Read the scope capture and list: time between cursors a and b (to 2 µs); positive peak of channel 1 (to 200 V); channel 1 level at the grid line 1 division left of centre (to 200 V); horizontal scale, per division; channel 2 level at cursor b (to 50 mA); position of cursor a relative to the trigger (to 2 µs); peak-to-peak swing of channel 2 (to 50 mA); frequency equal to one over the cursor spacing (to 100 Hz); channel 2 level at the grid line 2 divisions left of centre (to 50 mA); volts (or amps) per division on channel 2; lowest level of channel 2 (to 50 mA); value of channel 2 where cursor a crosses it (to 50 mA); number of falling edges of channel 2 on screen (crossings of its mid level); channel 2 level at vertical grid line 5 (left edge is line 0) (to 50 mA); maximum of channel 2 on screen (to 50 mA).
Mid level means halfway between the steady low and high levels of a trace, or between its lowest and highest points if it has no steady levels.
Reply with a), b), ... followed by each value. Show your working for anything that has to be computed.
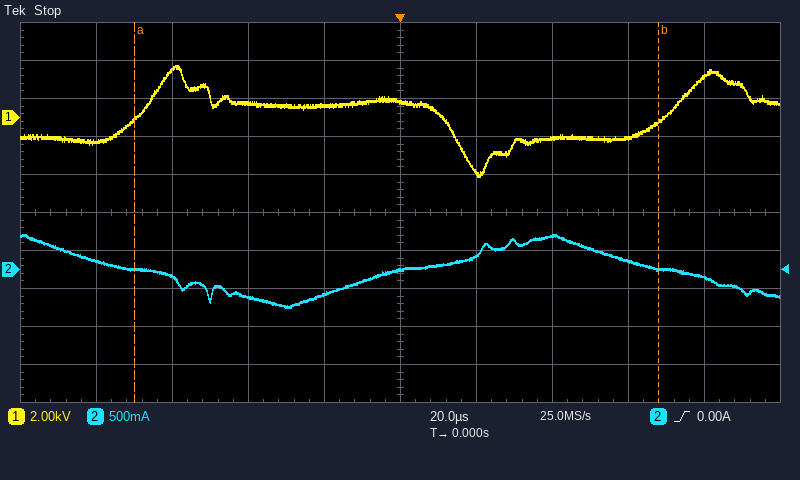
a) 138 µs
b) 2.8 kV
c) 600 V
d) 20 µs
e) 0 mA
f) -70 µs
g) 450 mA − (-500 mA) = 950 mA
h) 1 / 138 µs ≈ 7.2 kHz
i) -350 mA
j) 500 mA
k) -500 mA
l) 0 mA
m) 2
n) 0 mA
o) 450 mA
